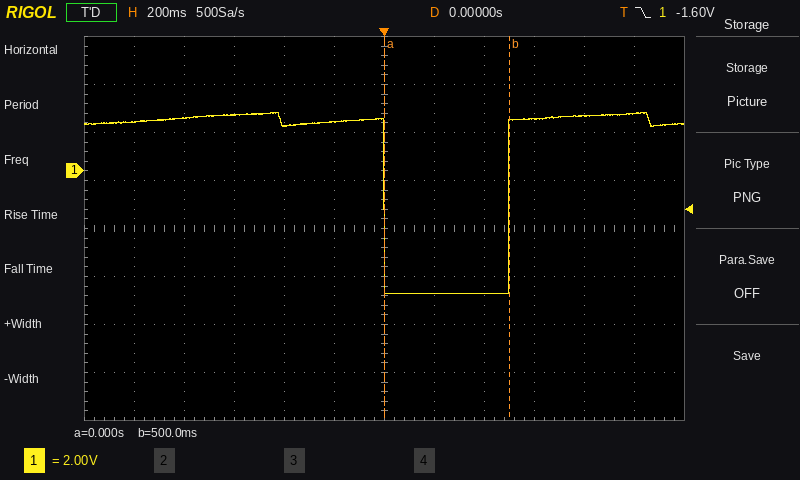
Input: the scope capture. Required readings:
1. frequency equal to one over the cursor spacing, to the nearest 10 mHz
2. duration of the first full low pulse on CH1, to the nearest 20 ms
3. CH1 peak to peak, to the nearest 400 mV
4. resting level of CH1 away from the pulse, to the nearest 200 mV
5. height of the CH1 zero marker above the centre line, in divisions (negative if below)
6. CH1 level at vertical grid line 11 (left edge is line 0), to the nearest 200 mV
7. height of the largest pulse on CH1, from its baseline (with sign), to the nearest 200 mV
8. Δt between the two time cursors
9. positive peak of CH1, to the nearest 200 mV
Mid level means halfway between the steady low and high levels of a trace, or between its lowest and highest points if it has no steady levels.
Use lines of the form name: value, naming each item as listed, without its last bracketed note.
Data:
frequency equal to one over the cursor spacing, to the nearest 10 mHz: 2.00 Hz
duration of the first full low pulse on CH1, to the nearest 20 ms: 500 ms
CH1 peak to peak, to the nearest 400 mV: 7.6 V
resting level of CH1 away from the pulse, to the nearest 200 mV: 2.2 V
height of the CH1 zero marker above the centre line, in divisions: +1.2 div
CH1 level at vertical grid line 11 (left edge is line 0), to the nearest 200 mV: 2.4 V
height of the largest pulse on CH1, from its baseline (with sign), to the nearest 200 mV: -7.2 V
Δt between the two time cursors: 500 ms
positive peak of CH1, to the nearest 200 mV: 2.4 V
